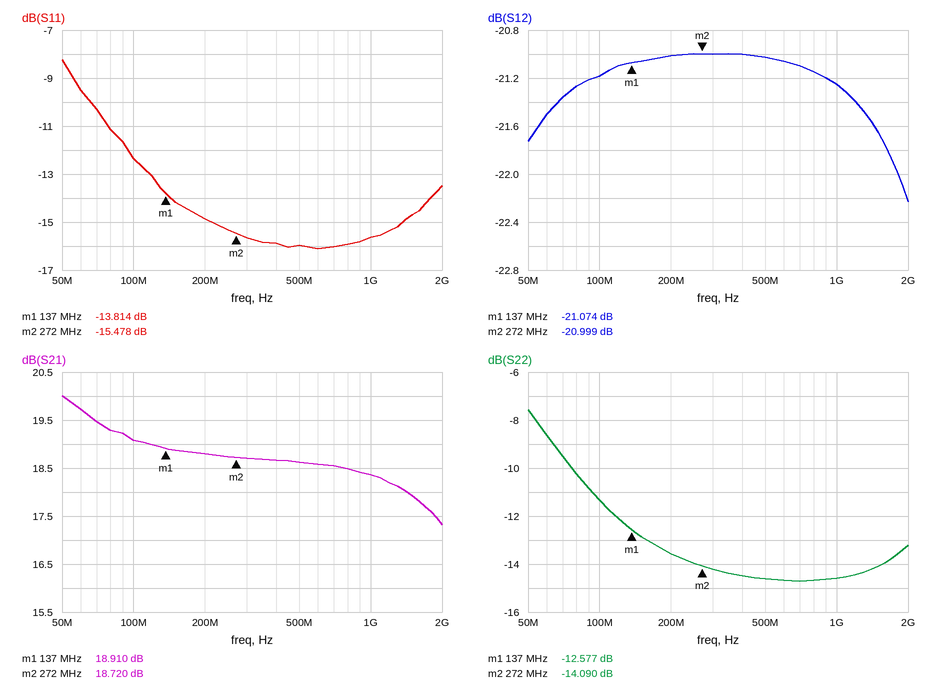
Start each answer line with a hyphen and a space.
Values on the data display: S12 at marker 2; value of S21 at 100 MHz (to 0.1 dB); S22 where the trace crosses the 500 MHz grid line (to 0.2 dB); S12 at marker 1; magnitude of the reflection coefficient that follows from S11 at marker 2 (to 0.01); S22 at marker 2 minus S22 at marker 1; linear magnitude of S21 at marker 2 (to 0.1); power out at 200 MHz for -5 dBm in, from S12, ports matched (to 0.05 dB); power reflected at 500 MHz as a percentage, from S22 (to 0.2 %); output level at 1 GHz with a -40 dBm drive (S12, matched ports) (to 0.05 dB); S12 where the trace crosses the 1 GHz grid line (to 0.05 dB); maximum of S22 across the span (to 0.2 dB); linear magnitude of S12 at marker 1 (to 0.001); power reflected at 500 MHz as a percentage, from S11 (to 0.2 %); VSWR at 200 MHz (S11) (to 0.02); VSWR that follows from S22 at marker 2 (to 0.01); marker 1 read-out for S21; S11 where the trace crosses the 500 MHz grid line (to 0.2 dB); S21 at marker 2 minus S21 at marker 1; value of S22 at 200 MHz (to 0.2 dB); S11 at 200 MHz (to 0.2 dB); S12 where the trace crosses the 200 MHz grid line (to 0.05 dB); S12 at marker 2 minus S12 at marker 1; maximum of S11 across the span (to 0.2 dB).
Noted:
- -20.999 dB
- 19.1 dB
- -14.6 dB
- -21.074 dB
- 0.17
- -1.513 dB
- 8.6
- -26.00 dBm
- 3.4 %
- -61.25 dBm
- -21.25 dB
- -7.6 dB
- 0.088
- 2.6 %
- 1.44
- 1.49
- 18.910 dB
- -16.0 dB
- -0.190 dB
- -13.6 dB
- -14.8 dB
- -21.00 dB
- 0.075 dB
- -8.2 dB
